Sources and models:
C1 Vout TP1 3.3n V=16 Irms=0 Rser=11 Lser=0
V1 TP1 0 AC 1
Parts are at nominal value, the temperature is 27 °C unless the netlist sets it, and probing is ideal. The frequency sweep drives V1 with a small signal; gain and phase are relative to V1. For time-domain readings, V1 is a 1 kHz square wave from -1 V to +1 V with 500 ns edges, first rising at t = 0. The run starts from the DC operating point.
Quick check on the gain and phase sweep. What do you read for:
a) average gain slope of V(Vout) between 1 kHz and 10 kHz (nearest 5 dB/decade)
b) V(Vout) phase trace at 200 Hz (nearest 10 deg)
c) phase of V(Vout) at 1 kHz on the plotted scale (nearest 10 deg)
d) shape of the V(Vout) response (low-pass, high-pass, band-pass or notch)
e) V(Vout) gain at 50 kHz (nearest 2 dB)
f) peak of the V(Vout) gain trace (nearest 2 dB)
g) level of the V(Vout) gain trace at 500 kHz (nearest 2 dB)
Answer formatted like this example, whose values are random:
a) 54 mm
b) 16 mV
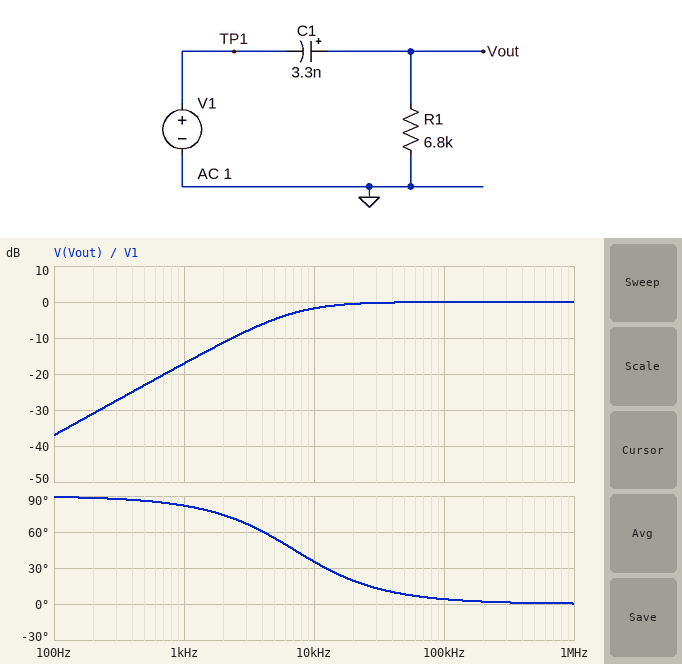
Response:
a) 15 dB/decade
b) 90 deg
c) 80 deg
d) high-pass
e) 0 dB
f) 0 dB
g) 0 dB
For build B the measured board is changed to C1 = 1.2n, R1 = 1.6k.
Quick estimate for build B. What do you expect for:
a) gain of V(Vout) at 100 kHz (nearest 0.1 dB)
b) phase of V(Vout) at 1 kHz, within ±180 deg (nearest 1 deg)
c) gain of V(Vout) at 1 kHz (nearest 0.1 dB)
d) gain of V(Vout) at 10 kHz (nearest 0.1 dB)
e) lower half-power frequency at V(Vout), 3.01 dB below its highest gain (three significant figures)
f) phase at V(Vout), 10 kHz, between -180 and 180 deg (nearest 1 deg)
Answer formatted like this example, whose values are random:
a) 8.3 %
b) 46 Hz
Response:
a) -2.3 dB
b) 89 deg
c) -38.4 dB
d) -18.4 dB
e) 82.3 kHz
f) 83 deg
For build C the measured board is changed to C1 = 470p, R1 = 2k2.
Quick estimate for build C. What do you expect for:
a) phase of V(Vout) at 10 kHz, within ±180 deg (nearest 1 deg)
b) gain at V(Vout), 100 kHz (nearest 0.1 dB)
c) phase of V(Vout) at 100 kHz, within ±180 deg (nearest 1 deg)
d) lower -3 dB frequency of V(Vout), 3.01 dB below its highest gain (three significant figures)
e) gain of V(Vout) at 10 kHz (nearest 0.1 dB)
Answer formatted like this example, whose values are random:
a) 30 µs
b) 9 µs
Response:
a) 86 deg
b) -5.3 dB
c) 57 deg
d) 153 kHz
e) -23.8 dB
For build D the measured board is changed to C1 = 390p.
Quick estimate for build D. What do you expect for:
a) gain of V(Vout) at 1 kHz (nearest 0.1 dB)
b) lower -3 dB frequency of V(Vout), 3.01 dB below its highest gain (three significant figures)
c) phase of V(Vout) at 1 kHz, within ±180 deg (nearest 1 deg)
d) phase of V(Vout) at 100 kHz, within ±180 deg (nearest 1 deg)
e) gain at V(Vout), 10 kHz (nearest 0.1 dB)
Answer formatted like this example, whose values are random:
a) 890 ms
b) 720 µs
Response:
a) -35.6 dB
b) 59.9 kHz
c) 89 deg
d) 31 deg
e) -15.7 dB
